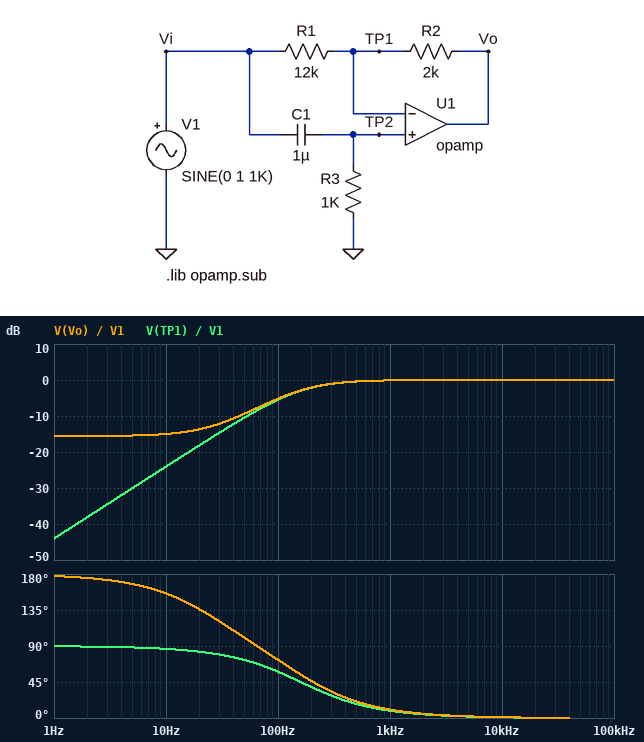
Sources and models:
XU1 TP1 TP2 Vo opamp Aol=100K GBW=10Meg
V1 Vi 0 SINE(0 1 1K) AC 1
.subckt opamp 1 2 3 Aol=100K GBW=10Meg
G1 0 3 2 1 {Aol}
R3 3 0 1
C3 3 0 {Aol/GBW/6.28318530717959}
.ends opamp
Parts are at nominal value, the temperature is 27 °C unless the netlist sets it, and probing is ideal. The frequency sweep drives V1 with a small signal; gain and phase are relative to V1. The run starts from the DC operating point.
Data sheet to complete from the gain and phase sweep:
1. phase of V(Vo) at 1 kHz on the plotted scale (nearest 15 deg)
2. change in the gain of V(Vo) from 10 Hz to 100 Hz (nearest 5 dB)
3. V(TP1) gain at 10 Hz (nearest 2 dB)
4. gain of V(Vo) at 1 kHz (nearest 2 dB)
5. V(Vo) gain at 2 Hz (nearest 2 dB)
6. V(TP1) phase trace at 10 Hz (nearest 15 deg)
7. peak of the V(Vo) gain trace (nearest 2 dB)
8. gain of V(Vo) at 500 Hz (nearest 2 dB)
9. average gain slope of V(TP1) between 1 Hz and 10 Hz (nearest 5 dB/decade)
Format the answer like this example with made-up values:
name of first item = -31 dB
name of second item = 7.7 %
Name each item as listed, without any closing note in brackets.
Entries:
phase of V(Vo) at 1 kHz on the plotted scale = 15 deg
change in the gain of V(Vo) from 10 Hz to 100 Hz = 10 dB
V(TP1) gain at 10 Hz = -24 dB
gain of V(Vo) at 1 kHz = 0 dB
V(Vo) gain at 2 Hz = -16 dB
V(TP1) phase trace at 10 Hz = 90 deg
peak of the V(Vo) gain trace = 0 dB
gain of V(Vo) at 500 Hz = 0 dB
average gain slope of V(TP1) between 1 Hz and 10 Hz = 20 dB/decade
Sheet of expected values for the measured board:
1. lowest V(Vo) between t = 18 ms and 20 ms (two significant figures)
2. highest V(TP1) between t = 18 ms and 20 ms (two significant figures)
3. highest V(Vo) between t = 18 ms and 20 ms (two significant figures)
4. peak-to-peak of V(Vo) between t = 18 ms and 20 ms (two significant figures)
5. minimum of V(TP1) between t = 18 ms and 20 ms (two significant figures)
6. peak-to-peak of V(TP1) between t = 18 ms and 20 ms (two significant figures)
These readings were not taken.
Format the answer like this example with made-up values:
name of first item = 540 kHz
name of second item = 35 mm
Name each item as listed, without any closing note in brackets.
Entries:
lowest V(Vo) between t = 18 ms and 20 ms = -990 mV
highest V(TP1) between t = 18 ms and 20 ms = 990 mV
highest V(Vo) between t = 18 ms and 20 ms = 990 mV
peak-to-peak of V(Vo) between t = 18 ms and 20 ms = 2.0 V
minimum of V(TP1) between t = 18 ms and 20 ms = -990 mV
peak-to-peak of V(TP1) between t = 18 ms and 20 ms = 2.0 V
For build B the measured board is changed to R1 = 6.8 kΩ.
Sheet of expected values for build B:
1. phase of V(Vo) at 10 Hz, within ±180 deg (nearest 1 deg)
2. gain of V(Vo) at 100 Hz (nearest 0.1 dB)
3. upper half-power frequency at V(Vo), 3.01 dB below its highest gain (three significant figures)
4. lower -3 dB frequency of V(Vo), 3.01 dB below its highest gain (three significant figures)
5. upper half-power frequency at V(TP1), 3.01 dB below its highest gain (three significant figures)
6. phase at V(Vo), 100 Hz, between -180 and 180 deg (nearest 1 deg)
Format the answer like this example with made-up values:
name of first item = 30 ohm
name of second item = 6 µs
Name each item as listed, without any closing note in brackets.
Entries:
phase of V(Vo) at 10 Hz, within ±180 deg = 164 deg
gain of V(Vo) at 100 Hz = -4.6 dB
upper half-power frequency at V(Vo), 3.01 dB below its highest gain = 7.73 MHz
lower -3 dB frequency of V(Vo), 3.01 dB below its highest gain = 145 Hz
upper half-power frequency at V(TP1), 3.01 dB below its highest gain = 8.16 MHz
phase at V(Vo), 100 Hz, between -180 and 180 deg = 83 deg
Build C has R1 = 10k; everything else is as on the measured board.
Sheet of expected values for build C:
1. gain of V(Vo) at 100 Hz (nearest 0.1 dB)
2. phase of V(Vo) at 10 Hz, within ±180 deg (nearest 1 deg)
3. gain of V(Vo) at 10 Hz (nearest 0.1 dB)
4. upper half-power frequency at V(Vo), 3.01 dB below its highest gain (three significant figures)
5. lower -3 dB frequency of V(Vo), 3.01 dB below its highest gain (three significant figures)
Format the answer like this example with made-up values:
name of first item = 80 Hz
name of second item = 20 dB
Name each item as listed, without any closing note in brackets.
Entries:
gain of V(Vo) at 100 Hz = -5.1 dB
phase of V(Vo) at 10 Hz, within ±180 deg = 159 deg
gain of V(Vo) at 10 Hz = -13.6 dB
upper half-power frequency at V(Vo), 3.01 dB below its highest gain = 8.33 MHz
lower -3 dB frequency of V(Vo), 3.01 dB below its highest gain = 153 Hz
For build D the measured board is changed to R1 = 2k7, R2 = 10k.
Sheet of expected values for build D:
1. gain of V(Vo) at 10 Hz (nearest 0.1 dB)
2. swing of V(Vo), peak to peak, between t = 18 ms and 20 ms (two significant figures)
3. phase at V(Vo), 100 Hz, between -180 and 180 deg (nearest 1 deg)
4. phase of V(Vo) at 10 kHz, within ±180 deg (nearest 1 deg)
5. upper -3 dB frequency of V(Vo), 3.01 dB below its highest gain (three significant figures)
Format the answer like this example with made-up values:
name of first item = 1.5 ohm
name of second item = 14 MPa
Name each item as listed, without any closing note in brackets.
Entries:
gain of V(Vo) at 10 Hz = 11.4 dB
swing of V(Vo), peak to peak, between t = 18 ms and 20 ms = 2.3 V
phase at V(Vo), 100 Hz, between -180 and 180 deg = 138 deg
phase of V(Vo) at 10 kHz, within ±180 deg = 4 deg
upper -3 dB frequency of V(Vo), 3.01 dB below its highest gain = 172 Hz
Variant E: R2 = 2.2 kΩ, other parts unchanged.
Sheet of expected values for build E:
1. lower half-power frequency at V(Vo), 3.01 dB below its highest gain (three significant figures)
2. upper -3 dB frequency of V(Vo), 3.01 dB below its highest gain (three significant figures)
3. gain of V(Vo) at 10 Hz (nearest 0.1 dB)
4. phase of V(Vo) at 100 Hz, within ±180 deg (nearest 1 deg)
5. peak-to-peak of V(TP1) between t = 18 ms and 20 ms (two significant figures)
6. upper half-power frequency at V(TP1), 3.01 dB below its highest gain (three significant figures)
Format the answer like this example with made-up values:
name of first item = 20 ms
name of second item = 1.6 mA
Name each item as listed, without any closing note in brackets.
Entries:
lower half-power frequency at V(Vo), 3.01 dB below its highest gain = 154 Hz
upper -3 dB frequency of V(Vo), 3.01 dB below its highest gain = 8.45 MHz
gain of V(Vo) at 10 Hz = -14.3 dB
phase of V(Vo) at 100 Hz, within ±180 deg = 74 deg
peak-to-peak of V(TP1) between t = 18 ms and 20 ms = 2.0 V
upper half-power frequency at V(TP1), 3.01 dB below its highest gain = 8.66 MHz
